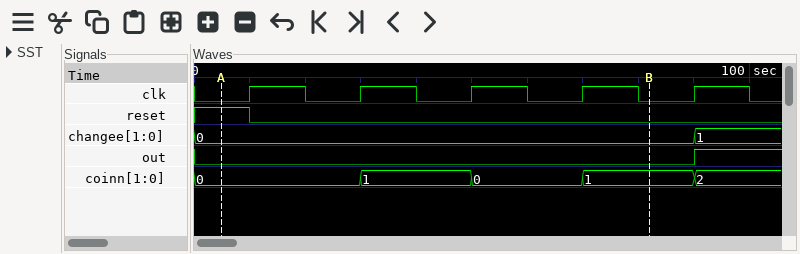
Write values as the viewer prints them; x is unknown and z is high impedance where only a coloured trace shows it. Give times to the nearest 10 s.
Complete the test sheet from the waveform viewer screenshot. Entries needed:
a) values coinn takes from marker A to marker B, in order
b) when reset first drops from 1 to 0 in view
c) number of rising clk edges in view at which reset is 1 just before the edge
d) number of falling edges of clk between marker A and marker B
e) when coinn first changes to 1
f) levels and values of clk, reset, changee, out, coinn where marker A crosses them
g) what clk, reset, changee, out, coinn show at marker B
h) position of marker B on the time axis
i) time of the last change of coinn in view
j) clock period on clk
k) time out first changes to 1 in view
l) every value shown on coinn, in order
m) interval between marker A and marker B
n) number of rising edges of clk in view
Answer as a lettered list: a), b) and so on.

a) 0, 1, 0, 1
b) 10 s
c) 1
d) 4
e) 30 s
f) clk=0, reset=1, changee=0, out=0, coinn=0
g) clk=0, reset=0, changee=0, out=0, coinn=1
h) 80 s
i) 90 s
j) 20 s
k) 90 s
l) 0, 1, 0, 1, 2
m) 80 s
n) 5
